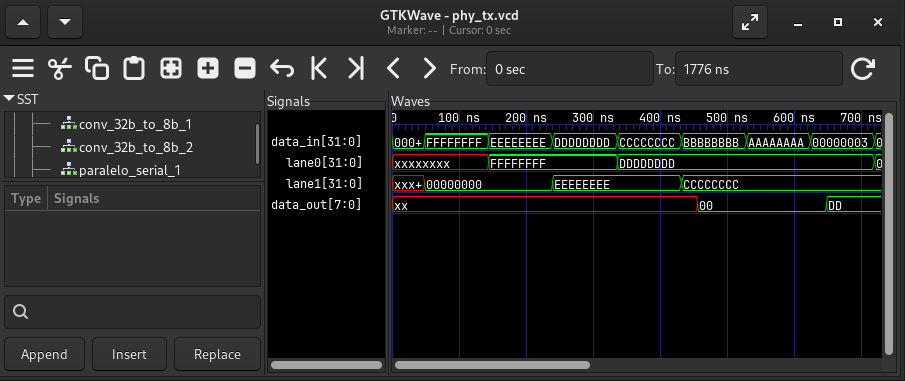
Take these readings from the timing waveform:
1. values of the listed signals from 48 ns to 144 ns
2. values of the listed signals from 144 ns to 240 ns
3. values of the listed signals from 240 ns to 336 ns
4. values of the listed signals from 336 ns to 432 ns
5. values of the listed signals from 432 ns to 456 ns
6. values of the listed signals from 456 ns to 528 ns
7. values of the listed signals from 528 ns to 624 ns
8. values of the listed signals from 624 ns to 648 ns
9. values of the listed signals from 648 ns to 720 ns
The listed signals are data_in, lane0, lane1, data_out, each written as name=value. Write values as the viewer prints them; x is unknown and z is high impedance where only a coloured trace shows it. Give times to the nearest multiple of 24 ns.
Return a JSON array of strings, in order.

["data_in=FFFFFFFF, lane0=xxxxxxxx, lane1=00000000, data_out=xx", "data_in=EEEEEEEE, lane0=FFFFFFFF, lane1=00000000, data_out=xx", "data_in=DDDDDDDD, lane0=FFFFFFFF, lane1=EEEEEEEE, data_out=xx", "data_in=CCCCCCCC, lane0=DDDDDDDD, lane1=EEEEEEEE, data_out=xx", "data_in=BBBBBBBB, lane0=DDDDDDDD, lane1=CCCCCCCC, data_out=xx", "data_in=BBBBBBBB, lane0=DDDDDDDD, lane1=CCCCCCCC, data_out=00", "data_in=AAAAAAAA, lane0=DDDDDDDD, lane1=CCCCCCCC, data_out=00", "data_in=00000003, lane0=DDDDDDDD, lane1=CCCCCCCC, data_out=00", "data_in=00000003, lane0=DDDDDDDD, lane1=CCCCCCCC, data_out=DD"]
